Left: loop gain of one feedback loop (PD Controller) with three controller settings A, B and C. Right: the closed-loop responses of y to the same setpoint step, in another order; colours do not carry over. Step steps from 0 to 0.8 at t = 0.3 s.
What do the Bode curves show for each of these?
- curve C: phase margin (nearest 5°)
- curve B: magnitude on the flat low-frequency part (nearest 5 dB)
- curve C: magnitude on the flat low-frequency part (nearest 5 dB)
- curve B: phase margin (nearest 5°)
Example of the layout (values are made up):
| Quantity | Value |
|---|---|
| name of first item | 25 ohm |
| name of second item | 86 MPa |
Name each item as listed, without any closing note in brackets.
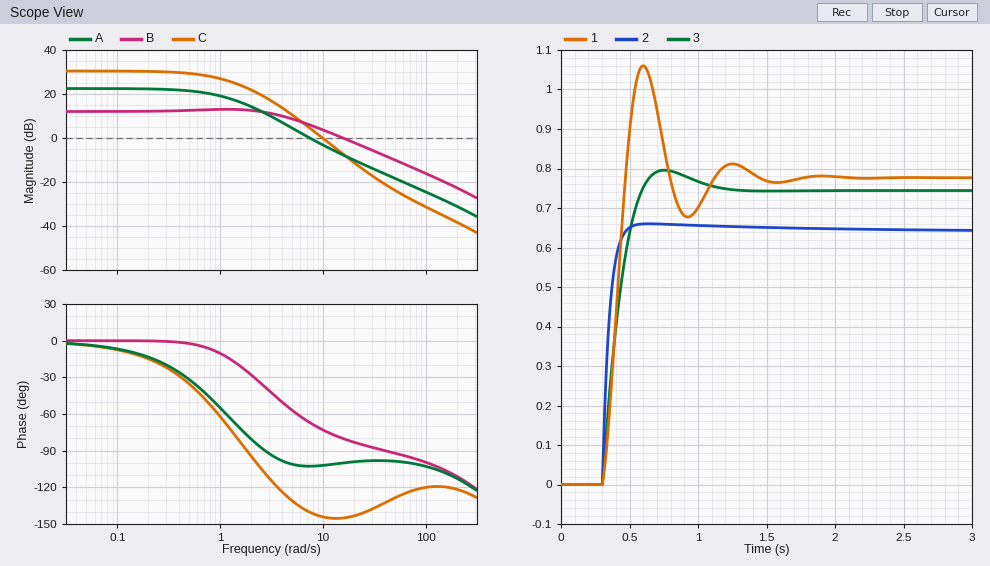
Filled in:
| Quantity | Value |
|---|---|
| curve C: phase margin | 35° |
| curve B: magnitude on the flat low-frequency part | 10 dB |
| curve C: magnitude on the flat low-frequency part | 30 dB |
| curve B: phase margin | 100° |
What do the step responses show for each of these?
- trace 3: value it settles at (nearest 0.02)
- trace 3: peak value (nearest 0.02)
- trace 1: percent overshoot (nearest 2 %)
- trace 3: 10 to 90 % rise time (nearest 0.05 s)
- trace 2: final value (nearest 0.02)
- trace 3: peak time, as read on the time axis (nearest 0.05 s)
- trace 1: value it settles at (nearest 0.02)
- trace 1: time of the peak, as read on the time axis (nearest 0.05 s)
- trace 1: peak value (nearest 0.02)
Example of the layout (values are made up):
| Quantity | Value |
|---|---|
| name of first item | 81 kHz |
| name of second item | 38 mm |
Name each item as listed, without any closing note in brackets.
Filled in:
| Quantity | Value |
|---|---|
| trace 3: value it settles at | 0.74 |
| trace 3: peak value | 0.80 |
| trace 1: percent overshoot | 36 % |
| trace 3: 10 to 90 % rise time | 0.20 s |
| trace 2: final value | 0.64 |
| trace 3: peak time, as read on the time axis | 0.75 s |
| trace 1: value it settles at | 0.78 |
| trace 1: time of the peak, as read on the time axis | 0.60 s |
| trace 1: peak value | 1.06 |
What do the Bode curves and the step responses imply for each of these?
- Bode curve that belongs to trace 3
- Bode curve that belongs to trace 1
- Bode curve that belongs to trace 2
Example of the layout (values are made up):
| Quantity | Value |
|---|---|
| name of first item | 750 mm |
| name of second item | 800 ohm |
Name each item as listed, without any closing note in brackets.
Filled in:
| Quantity | Value |
|---|---|
| Bode curve that belongs to trace 3 | A |
| Bode curve that belongs to trace 1 | C |
| Bode curve that belongs to trace 2 | B |
